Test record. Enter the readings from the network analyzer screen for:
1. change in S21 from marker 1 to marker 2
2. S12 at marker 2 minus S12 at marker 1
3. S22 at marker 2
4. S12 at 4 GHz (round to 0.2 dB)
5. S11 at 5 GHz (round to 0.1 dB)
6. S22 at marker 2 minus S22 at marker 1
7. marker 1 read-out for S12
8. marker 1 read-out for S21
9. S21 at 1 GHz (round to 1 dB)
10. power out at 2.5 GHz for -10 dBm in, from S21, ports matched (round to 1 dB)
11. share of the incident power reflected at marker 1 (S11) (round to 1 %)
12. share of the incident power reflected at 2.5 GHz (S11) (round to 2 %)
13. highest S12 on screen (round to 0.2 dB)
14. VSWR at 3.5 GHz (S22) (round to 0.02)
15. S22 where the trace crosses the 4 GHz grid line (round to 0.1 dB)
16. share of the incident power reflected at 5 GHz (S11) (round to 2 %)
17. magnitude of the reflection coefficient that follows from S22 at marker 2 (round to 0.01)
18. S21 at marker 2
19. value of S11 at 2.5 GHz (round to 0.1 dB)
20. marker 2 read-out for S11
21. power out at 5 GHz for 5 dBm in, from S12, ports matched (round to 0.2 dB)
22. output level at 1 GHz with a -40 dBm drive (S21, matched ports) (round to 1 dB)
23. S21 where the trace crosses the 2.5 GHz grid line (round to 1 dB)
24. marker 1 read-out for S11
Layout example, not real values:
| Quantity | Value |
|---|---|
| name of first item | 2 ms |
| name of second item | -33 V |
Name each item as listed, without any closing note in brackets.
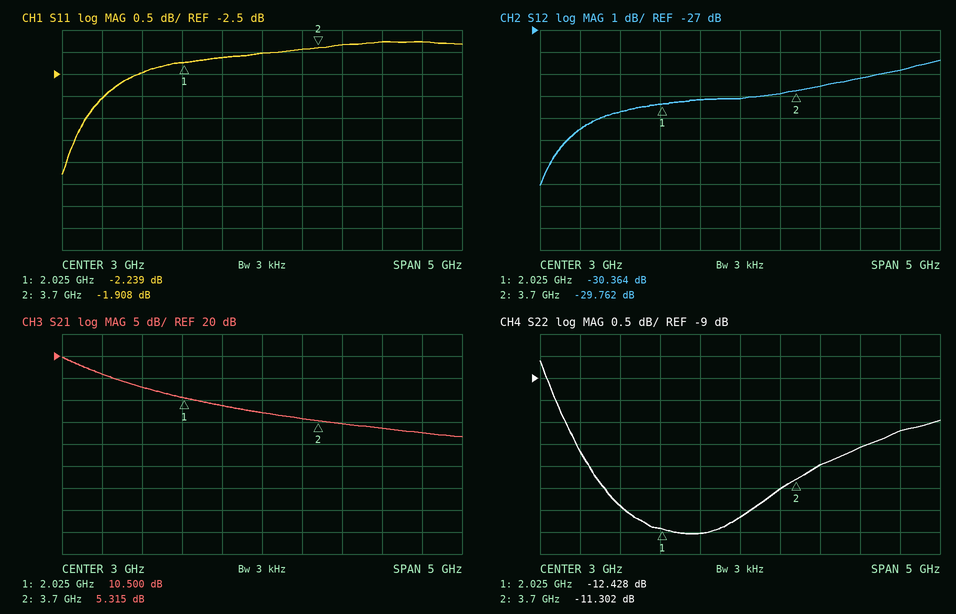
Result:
| Quantity | Value |
|---|---|
| change in S21 from marker 1 to marker 2 | -5.185 dB |
| S12 at marker 2 minus S12 at marker 1 | 0.602 dB |
| S22 at marker 2 | -11.302 dB |
| S12 at 4 GHz | -29.6 dB |
| S11 at 5 GHz | -1.8 dB |
| S22 at marker 2 minus S22 at marker 1 | 1.126 dB |
| marker 1 read-out for S12 | -30.364 dB |
| marker 1 read-out for S21 | 10.500 dB |
| S21 at 1 GHz | 16 dB |
| power out at 2.5 GHz for -10 dBm in, from S21, ports matched | -1 dBm |
| share of the incident power reflected at marker 1 (S11) | 60 % |
| share of the incident power reflected at 2.5 GHz (S11) | 62 % |
| highest S12 on screen | -28.4 dB |
| VSWR at 3.5 GHz (S22) | 1.72 |
| S22 where the trace crosses the 4 GHz grid line | -11.0 dB |
| share of the incident power reflected at 5 GHz (S11) | 66 % |
| magnitude of the reflection coefficient that follows from S22 at marker 2 | 0.27 |
| S21 at marker 2 | 5.315 dB |
| value of S11 at 2.5 GHz | -2.1 dB |
| marker 2 read-out for S11 | -1.908 dB |
| power out at 5 GHz for 5 dBm in, from S12, ports matched | -23.8 dBm |
| output level at 1 GHz with a -40 dBm drive (S21, matched ports) | -24 dBm |
| S21 where the trace crosses the 2.5 GHz grid line | 9 dB |
| marker 1 read-out for S11 | -2.239 dB |
